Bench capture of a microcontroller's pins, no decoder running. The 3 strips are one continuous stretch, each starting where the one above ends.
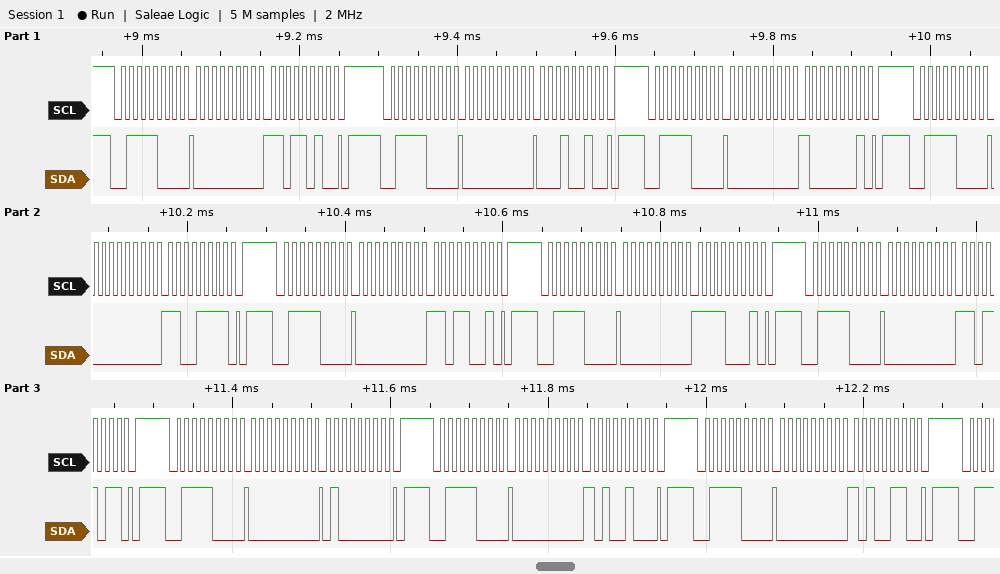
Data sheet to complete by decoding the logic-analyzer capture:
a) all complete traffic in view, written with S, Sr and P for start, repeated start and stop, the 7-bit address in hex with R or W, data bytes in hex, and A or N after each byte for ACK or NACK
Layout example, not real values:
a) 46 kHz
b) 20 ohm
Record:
a) S 3CW A 00 A DA A P S 3CW A 00 A 12 A P S 3CW A 00 A 81 A P S 3CW A 00 A CF A P S 3CW A 00 A D9 A P S 3CW A 00 A F1 A P S 3CW A 00 A DB A P S 3CW A 00 A 40 A P S 3CW A 00 A A4 A P S 3CW A 00 A A6 A P
